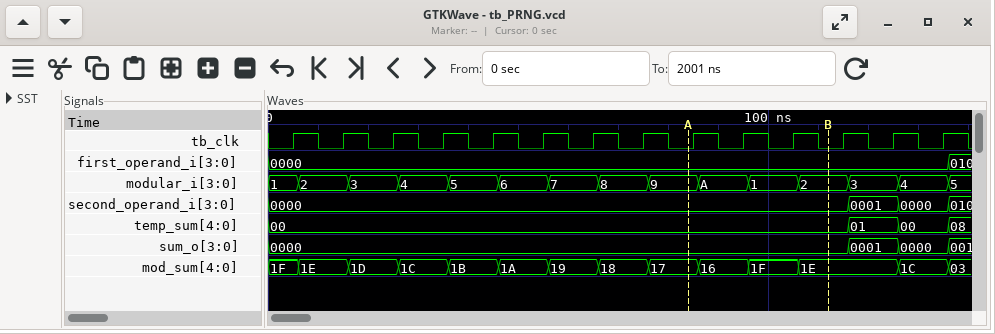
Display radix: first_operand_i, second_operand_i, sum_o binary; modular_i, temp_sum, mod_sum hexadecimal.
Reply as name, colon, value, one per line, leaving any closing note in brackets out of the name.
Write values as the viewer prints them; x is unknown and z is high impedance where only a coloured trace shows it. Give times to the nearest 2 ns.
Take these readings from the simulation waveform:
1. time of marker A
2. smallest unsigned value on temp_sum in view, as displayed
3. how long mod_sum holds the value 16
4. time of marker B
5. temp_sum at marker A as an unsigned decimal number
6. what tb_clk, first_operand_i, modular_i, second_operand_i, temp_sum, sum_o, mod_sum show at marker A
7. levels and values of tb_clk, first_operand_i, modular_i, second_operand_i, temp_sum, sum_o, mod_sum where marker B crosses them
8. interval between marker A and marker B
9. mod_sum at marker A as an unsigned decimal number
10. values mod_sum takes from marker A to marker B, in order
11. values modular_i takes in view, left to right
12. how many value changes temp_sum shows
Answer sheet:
time of marker A: 84 ns
smallest unsigned value on temp_sum in view, as displayed: 00
how long mod_sum holds the value 16: 10 ns
time of marker B: 112 ns
temp_sum at marker A as an unsigned decimal number: 0
what tb_clk, first_operand_i, modular_i, second_operand_i, temp_sum, sum_o, mod_sum show at marker A: tb_clk=0, first_operand_i=0000, modular_i=9, second_operand_i=0000, temp_sum=00, sum_o=0000, mod_sum=17
levels and values of tb_clk, first_operand_i, modular_i, second_operand_i, temp_sum, sum_o, mod_sum where marker B crosses them: tb_clk=0, first_operand_i=0000, modular_i=2, second_operand_i=0000, temp_sum=00, sum_o=0000, mod_sum=1E
interval between marker A and marker B: 28 ns
mod_sum at marker A as an unsigned decimal number: 23
values mod_sum takes from marker A to marker B, in order: 17, 16, 1F, 1E
values modular_i takes in view, left to right: 1, 2, 3, 4, 5, 6, 7, 8, 9, A, 1, 2, 3, 4, 5
how many value changes temp_sum shows: 3
